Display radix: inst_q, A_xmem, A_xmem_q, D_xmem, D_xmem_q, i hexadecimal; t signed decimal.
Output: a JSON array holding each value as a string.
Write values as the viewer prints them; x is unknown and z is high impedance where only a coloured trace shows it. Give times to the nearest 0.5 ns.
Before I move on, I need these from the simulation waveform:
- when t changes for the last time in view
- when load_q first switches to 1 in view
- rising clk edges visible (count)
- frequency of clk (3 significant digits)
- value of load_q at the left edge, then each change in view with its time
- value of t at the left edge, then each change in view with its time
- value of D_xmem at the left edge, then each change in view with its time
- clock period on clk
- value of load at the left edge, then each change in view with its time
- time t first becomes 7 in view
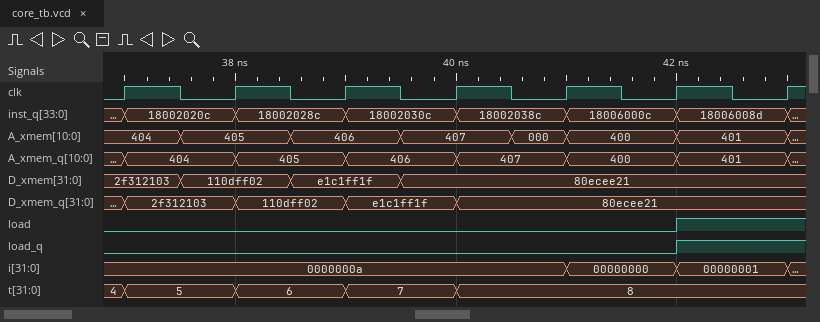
["40 ns", "42 ns", "7", "1.00 GHz", "0, 1 at 42 ns", "4, 5 at 37 ns, 6 at 38 ns, 7 at 39 ns, 8 at 40 ns", "2f312103, 110dff02 at 37.5 ns, e1c1ff1f at 38.5 ns, 80ecee21 at 39.5 ns", "1 ns", "0, 1 at 42 ns", "39 ns"]
